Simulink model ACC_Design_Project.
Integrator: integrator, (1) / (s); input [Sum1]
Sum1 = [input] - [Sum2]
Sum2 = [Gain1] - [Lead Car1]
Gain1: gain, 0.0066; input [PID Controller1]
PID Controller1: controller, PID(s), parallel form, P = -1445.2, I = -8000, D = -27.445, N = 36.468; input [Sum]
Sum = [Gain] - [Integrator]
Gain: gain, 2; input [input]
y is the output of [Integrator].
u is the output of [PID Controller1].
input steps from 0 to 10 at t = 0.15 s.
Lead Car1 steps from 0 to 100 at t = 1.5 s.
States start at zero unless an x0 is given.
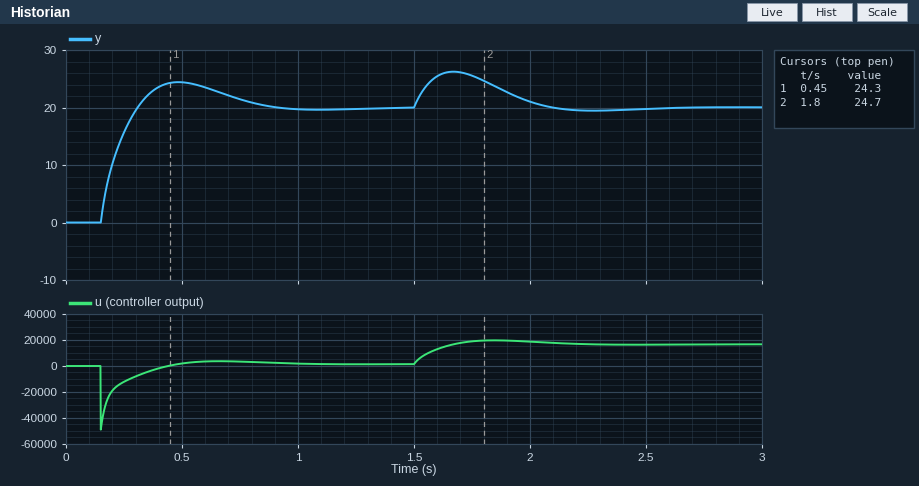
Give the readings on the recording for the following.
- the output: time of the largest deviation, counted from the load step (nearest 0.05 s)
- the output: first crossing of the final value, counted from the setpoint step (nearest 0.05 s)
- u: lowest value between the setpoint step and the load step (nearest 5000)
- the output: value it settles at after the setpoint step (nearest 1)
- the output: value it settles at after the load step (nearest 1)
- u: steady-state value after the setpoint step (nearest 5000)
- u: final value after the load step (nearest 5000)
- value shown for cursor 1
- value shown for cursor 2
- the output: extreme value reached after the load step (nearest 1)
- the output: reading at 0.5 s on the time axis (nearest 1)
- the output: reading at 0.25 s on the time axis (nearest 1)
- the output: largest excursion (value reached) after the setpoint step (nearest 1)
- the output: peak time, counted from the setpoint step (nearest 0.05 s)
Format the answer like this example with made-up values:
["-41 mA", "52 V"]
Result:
["0.15 s", "0.15 s", "-50000", "20", "20", "0", "15000", "24.3", "24.7", "26", "24", "16", "24", "0.35 s"]
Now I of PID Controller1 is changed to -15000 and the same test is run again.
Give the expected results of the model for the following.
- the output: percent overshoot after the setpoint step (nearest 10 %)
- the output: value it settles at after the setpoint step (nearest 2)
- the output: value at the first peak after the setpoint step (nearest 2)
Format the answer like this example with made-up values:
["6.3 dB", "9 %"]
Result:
["30 %", "20", "26"]
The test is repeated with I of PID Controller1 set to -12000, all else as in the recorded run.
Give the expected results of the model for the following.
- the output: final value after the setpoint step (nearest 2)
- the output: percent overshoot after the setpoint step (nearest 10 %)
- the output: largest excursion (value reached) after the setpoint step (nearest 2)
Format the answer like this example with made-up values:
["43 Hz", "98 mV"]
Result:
["20", "30 %", "26"]
